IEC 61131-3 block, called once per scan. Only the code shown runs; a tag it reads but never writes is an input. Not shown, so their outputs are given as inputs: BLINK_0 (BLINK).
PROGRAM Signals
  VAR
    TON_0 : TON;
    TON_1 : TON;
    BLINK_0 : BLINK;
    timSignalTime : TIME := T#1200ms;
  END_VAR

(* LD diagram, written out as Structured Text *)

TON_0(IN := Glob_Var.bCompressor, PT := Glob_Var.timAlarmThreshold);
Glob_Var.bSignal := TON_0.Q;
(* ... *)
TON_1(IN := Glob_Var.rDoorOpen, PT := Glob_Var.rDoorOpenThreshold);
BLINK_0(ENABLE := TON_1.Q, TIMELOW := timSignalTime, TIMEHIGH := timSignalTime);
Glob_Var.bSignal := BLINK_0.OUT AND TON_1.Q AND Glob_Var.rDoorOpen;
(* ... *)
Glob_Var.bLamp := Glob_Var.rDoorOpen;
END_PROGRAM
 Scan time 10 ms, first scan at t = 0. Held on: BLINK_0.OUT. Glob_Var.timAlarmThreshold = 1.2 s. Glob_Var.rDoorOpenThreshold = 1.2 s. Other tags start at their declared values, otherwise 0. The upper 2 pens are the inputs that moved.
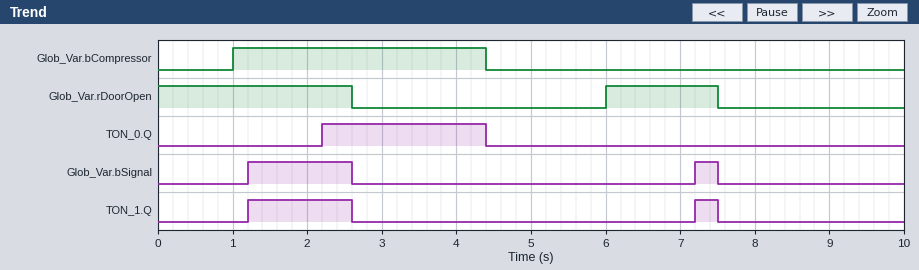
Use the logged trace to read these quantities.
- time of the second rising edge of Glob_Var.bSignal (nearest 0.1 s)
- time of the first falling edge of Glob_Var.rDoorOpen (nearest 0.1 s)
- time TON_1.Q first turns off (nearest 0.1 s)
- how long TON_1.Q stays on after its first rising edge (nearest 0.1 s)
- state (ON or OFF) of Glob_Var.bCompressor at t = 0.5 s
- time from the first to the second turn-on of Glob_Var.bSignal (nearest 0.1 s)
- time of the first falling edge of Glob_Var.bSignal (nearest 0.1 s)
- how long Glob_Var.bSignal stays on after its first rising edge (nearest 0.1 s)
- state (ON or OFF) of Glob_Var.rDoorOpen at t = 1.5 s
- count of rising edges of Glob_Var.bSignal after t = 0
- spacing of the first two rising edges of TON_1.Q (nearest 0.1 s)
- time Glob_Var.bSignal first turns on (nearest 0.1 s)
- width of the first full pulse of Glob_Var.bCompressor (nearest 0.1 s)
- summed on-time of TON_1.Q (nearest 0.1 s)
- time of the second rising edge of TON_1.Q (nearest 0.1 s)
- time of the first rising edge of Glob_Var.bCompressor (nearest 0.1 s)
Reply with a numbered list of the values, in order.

1. 7.2 s
2. 2.6 s
3. 2.6 s
4. 1.4 s
5. OFF
6. 6.0 s
7. 2.6 s
8. 1.4 s
9. ON
10. 2
11. 6.0 s
12. 1.2 s
13. 3.4 s
14. 1.7 s
15. 7.2 s
16. 1.0 s
